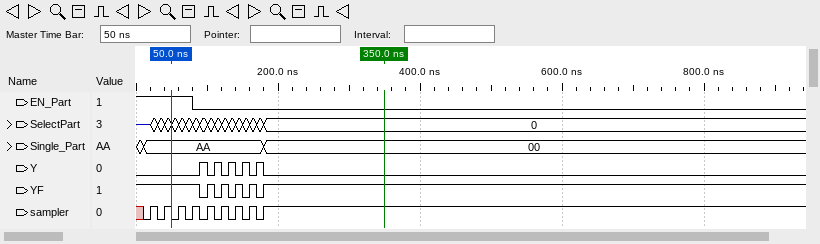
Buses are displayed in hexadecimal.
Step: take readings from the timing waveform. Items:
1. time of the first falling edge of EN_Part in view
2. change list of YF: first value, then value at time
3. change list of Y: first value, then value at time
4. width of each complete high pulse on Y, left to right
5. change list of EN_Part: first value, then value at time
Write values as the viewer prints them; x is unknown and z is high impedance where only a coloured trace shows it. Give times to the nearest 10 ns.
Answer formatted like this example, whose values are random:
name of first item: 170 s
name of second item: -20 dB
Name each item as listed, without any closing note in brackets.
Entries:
time of the first falling edge of EN_Part in view: 80 ns
change list of YF: first value, then value at time: 1, 0 at 90 ns, 1 at 100 ns, 0 at 110 ns, 1 at 120 ns, 0 at 130 ns, 1 at 140 ns, 0 at 150 ns, 1 at 160 ns, 0 at 170 ns, 1 at 180 ns
change list of Y: first value, then value at time: 0, 1 at 90 ns, 0 at 100 ns, 1 at 110 ns, 0 at 120 ns, 1 at 130 ns, 0 at 140 ns, 1 at 150 ns, 0 at 160 ns, 1 at 170 ns, 0 at 180 ns
width of each complete high pulse on Y, left to right: 10 ns, 10 ns, 10 ns, 10 ns, 10 ns
change list of EN_Part: first value, then value at time: 1, 0 at 80 ns
